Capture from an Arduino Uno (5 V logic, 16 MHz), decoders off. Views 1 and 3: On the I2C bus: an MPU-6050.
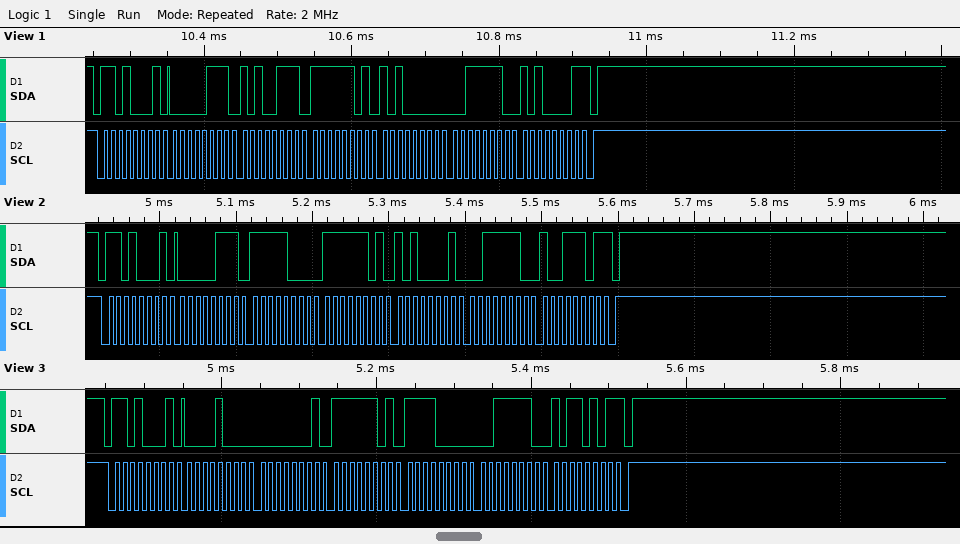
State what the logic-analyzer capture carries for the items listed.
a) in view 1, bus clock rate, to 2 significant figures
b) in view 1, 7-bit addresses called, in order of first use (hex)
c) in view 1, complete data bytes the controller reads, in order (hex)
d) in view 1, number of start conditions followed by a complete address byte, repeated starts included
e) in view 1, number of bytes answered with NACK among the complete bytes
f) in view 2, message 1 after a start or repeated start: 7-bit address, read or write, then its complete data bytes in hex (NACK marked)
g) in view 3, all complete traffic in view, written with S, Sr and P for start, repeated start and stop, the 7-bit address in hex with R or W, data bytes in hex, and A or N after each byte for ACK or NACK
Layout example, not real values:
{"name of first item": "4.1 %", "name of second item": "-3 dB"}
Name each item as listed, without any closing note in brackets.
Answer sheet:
{"in view 1, bus clock rate, to 2 significant figures": "100 kHz", "in view 1, 7-bit addresses called, in order of first use": "0x68", "in view 1, complete data bytes the controller reads, in order": "07 A7 FD A0 3E A1", "in view 1, number of start conditions followed by a complete address byte, repeated starts included": "1", "in view 1, number of bytes answered with NACK among the complete bytes": "1", "in view 2, message 1 after a start or repeated start: 7-bit address, read or write, then its complete data bytes in hex": "0x68 read: 07 F8 FD A1 3E 9D NACK", "in view 3, all complete traffic in view, written with S, Sr and P for start, repeated start and stop, the 7-bit address in hex with R or W, data bytes in hex, and A or N after each byte for ACK or NACK": "S 68R A 08 A 01 A FD A F0 A 3E A B5 N P"}
